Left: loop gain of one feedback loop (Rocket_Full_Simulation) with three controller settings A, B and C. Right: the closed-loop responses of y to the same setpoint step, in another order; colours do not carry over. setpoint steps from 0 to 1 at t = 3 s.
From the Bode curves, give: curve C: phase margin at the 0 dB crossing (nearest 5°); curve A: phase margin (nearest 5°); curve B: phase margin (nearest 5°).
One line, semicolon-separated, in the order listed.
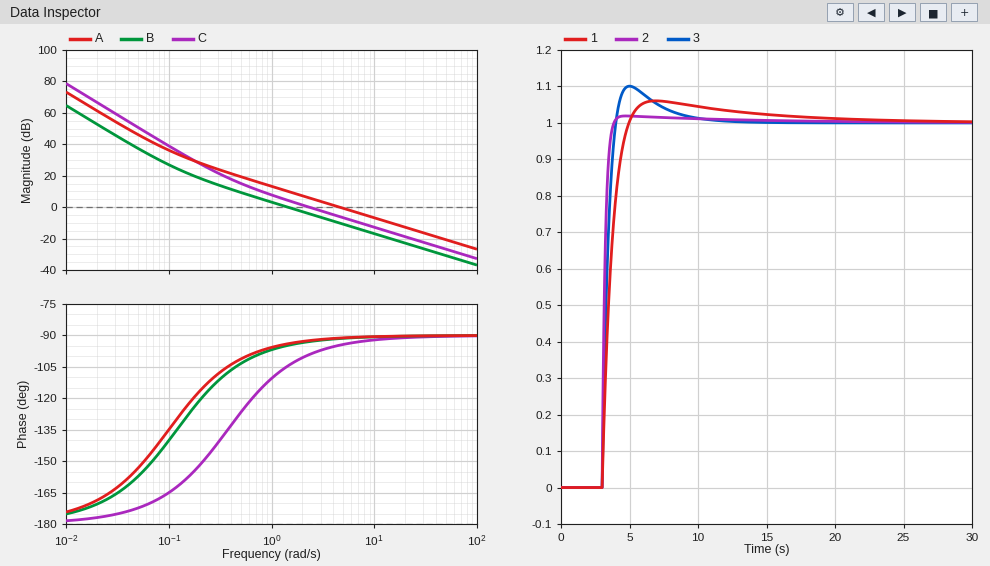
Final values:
80°; 90°; 85°
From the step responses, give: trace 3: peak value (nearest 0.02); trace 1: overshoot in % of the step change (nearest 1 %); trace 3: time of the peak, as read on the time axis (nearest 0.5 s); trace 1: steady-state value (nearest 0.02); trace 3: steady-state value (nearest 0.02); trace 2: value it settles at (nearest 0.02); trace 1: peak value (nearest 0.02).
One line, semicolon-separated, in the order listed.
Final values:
1.10; 6 %; 5.0 s; 1.00; 1.00; 1.00; 1.06
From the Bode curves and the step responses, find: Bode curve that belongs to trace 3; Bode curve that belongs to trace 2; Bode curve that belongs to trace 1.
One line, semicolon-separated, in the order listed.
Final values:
C; A; B
